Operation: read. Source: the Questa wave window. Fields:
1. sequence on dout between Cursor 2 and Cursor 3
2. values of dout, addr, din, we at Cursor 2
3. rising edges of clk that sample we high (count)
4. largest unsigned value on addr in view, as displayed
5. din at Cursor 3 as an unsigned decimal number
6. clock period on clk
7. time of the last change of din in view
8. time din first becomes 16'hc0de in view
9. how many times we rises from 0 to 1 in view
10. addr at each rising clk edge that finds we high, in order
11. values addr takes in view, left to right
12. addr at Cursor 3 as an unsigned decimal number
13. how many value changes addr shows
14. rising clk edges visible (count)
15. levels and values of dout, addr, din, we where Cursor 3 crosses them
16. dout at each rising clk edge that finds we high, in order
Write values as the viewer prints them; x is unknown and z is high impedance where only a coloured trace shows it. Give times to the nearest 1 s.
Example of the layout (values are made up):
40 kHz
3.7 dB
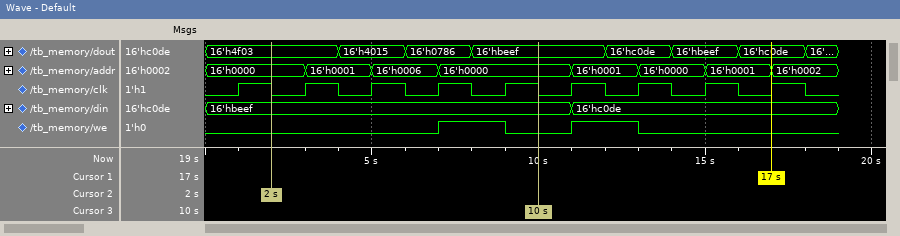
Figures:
16'h4f03, 16'h4015, 16'h0786, 16'hbeef
dout=16'h4f03, addr=16'h0000, din=16'hbeef, we=0
2
16'h0006
48879
2 s
11 s
11 s
2
16'h0000, 16'h0001
16'h0000, 16'h0001, 16'h0006, 16'h0000, 16'h0001, 16'h0000, 16'h0001, 16'h0002
0
7
9
dout=16'hbeef, addr=16'h0000, din=16'hbeef, we=0
16'hbeef, 16'hc0de
